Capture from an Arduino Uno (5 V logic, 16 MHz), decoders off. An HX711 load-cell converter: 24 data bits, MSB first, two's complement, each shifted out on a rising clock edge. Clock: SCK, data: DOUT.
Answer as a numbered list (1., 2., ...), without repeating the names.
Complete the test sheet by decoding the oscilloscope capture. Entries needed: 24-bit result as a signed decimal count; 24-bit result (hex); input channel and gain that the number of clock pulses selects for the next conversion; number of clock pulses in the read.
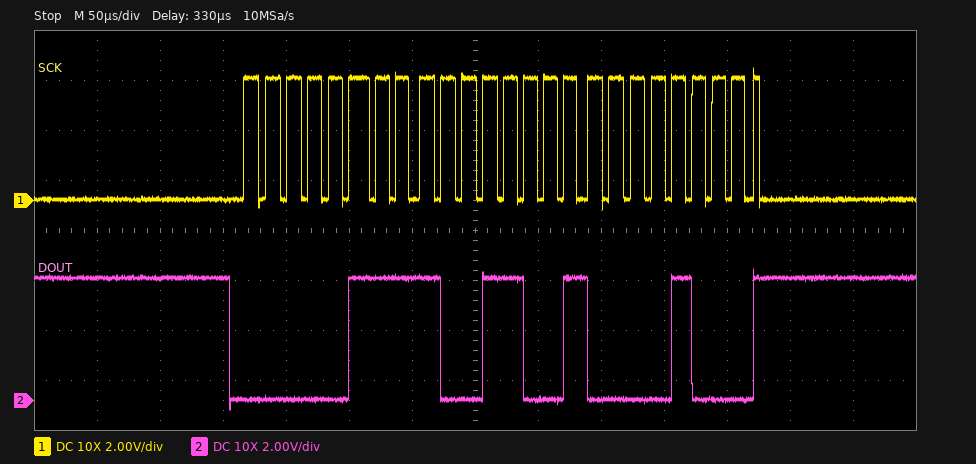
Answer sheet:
1. 497928
2. 0x079908
3. channel A, gain 128
4. 25
